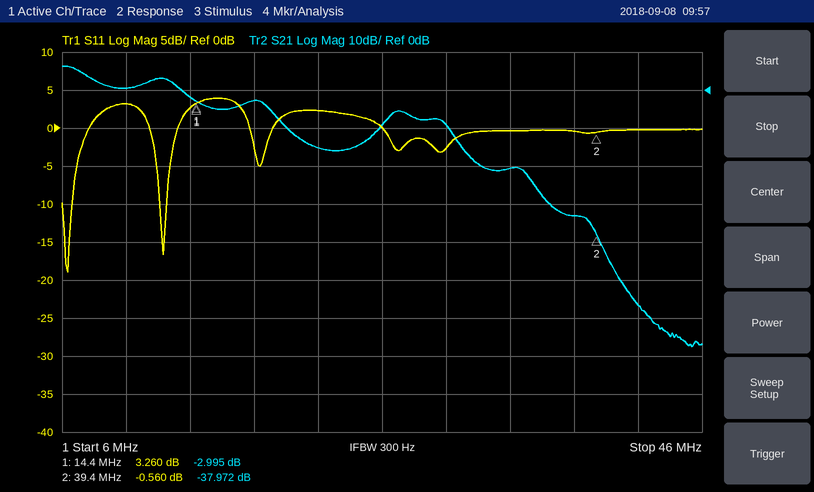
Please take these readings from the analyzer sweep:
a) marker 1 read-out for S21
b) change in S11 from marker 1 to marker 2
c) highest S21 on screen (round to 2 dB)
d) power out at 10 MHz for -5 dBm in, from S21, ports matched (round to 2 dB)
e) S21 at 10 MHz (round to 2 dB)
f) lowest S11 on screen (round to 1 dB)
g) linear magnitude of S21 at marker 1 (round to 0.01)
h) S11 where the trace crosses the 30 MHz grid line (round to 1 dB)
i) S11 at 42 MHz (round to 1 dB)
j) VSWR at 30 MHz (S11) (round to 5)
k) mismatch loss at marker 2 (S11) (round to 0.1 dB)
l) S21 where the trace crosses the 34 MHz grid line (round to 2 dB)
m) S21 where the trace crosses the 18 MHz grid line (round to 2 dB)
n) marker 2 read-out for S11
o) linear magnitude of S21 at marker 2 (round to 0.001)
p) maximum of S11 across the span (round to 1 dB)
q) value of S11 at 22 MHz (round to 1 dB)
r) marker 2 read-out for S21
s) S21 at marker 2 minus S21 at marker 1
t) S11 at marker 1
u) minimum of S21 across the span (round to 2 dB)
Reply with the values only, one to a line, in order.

-2.995 dB
-3.820 dB
6 dB
-4 dBm
0 dB
-19 dB
0.71
-3 dB
0 dB
5
9.2 dB
-20 dB
-2 dB
-0.560 dB
0.013
4 dB
2 dB
-37.972 dB
-34.977 dB
3.260 dB
-68 dB
